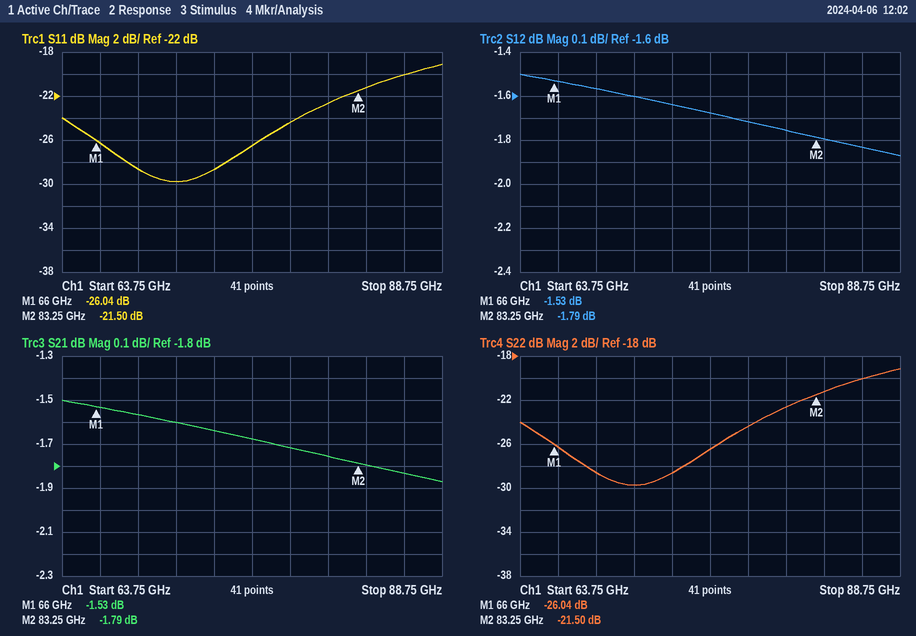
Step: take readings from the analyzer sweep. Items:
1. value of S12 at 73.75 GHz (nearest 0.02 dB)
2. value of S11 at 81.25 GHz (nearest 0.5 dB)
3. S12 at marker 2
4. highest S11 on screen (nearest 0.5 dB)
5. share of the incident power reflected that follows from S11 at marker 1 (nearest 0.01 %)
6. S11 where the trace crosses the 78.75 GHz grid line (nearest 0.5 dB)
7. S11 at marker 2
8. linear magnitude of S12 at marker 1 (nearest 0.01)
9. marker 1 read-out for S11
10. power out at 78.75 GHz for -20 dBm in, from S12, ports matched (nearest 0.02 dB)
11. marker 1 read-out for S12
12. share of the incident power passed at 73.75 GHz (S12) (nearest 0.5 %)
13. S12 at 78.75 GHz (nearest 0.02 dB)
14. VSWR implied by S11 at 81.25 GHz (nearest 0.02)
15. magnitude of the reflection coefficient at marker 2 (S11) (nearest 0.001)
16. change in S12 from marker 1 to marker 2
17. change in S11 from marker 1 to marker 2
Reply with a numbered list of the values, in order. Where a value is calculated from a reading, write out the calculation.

1. -1.64 dB
2. -22.5 dB
3. -1.79 dB
4. -19.0 dB
5. 10^(-26.04/10) ≈ 0.25 %
6. -24.5 dB
7. -21.50 dB
8. 10^(-1.53/20) ≈ 0.84
9. -26.04 dB
10. -20 dBm + (-1.72 dB) = -21.72 dBm
11. -1.53 dB
12. 10^(-1.64/10) ≈ 68.5 %
13. -1.72 dB
14. |Γ| = 10^(-22.5/20) = 0.0750; VSWR = (1 + 0.0750)/(1 − 0.0750) ≈ 1.16
15. 10^(-21.5/20) ≈ 0.084
16. -1.79 − (-1.53) = -0.26 dB
17. -21.5 − (-26.04) = 4.54 dB
